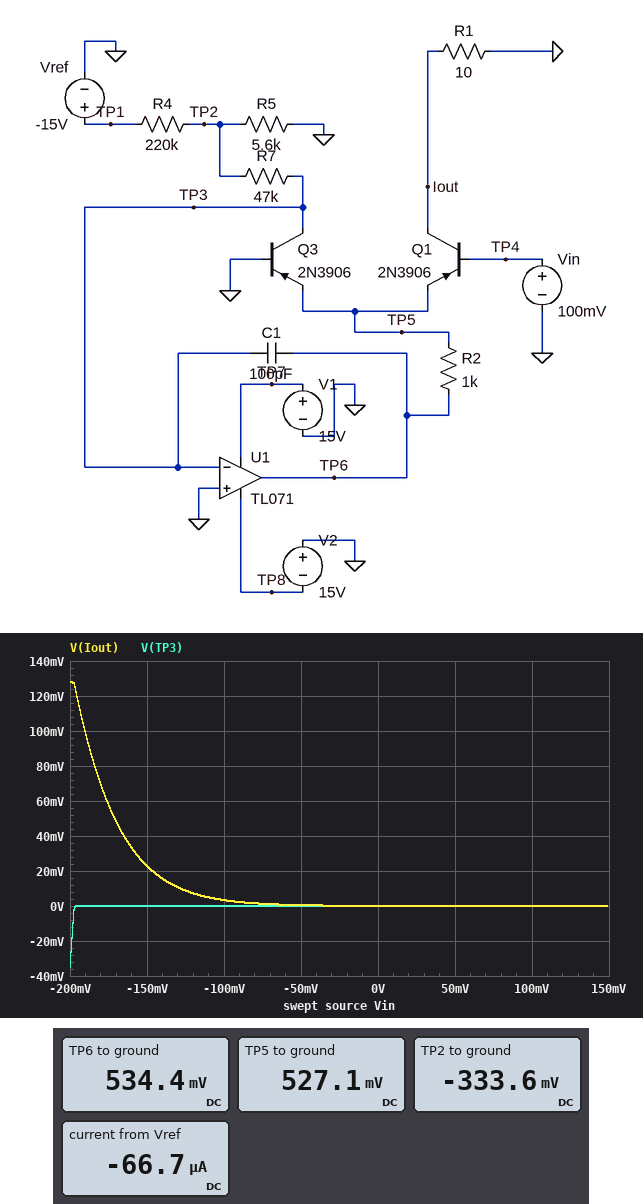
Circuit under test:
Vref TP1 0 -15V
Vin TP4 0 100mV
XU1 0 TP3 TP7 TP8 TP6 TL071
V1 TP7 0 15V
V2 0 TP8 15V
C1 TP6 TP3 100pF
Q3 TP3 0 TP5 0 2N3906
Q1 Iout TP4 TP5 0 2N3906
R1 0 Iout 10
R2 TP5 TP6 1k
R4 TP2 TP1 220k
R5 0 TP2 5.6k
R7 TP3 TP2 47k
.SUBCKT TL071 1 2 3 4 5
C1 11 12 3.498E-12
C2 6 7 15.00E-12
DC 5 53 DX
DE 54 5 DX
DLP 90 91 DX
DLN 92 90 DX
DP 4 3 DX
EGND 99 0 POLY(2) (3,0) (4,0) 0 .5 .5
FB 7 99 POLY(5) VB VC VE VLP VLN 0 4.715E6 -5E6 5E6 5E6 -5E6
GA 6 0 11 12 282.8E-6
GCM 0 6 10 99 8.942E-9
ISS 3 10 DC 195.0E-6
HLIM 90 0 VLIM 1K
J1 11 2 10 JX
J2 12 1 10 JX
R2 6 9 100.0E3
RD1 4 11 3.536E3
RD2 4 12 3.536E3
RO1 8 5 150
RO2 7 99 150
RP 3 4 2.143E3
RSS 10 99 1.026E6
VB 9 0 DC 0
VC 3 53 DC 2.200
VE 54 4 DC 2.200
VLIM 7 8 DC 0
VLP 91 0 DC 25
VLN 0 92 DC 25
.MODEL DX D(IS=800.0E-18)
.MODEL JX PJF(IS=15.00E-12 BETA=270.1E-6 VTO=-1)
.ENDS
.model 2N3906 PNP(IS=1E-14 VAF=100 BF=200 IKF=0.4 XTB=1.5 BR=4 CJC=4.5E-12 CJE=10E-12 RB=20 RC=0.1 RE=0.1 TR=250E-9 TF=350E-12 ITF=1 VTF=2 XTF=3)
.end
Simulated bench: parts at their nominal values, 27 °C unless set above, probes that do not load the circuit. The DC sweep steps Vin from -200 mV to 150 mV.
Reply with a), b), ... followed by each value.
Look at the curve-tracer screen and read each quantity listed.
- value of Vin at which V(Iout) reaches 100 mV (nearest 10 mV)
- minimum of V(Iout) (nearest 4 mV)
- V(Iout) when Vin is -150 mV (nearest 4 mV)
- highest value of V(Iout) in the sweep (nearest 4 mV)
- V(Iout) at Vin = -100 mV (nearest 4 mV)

a) -190 mV
b) 0 V
c) 24 mV
d) 128 mV
e) 4 mV
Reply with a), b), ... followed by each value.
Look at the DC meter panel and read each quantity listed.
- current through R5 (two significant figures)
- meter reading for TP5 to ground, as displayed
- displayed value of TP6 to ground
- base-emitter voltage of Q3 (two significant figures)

a) 60 µA
b) 527.1 mV
c) 534.4 mV
d) -530 mV
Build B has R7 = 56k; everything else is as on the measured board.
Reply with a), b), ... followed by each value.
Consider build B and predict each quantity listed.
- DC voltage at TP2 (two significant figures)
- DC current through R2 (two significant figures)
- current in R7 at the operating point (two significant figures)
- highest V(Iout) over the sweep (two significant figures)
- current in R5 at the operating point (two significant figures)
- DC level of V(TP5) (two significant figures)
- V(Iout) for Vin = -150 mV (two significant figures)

a) -340 mV
b) 6.2 µA
c) 6.1 µA
d) 120 mV
e) 61 µA
f) 520 mV
g) 20 mV
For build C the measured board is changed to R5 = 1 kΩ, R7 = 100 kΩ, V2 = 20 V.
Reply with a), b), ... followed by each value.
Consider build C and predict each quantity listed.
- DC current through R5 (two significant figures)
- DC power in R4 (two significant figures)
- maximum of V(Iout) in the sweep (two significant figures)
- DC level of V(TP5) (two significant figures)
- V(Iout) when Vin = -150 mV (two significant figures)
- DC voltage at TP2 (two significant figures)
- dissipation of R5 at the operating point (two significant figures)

a) 67 µA
b) 1.0 mW
c) 15 mV
d) 470 mV
e) 2.2 mV
f) -67 mV
g) 4.5 µW
